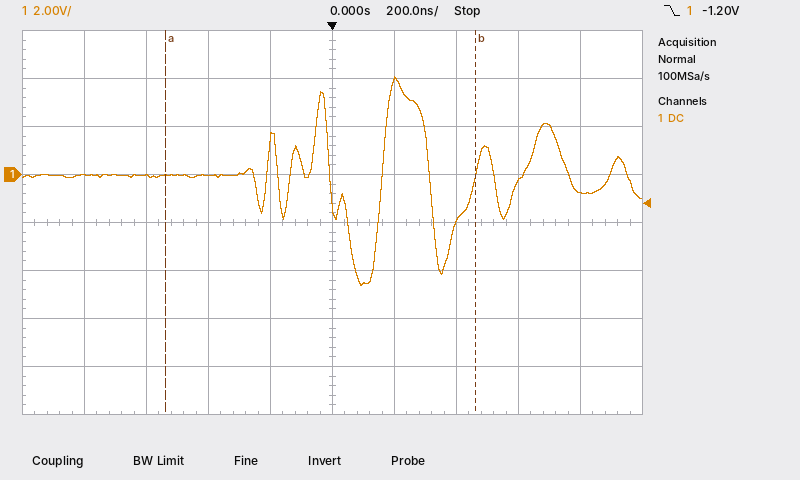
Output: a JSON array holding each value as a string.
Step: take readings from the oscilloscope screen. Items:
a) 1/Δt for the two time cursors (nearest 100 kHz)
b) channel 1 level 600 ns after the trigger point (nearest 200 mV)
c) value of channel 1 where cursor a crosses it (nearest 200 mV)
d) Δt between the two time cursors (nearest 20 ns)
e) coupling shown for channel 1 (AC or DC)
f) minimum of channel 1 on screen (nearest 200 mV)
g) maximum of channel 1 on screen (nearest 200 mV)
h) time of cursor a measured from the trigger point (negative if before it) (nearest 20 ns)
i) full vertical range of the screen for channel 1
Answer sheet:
["1.0 MHz", "-400 mV", "0.0 V", "1.00 µs", "DC", "-4.6 V", "4.0 V", "-540 ns", "16 V"]
